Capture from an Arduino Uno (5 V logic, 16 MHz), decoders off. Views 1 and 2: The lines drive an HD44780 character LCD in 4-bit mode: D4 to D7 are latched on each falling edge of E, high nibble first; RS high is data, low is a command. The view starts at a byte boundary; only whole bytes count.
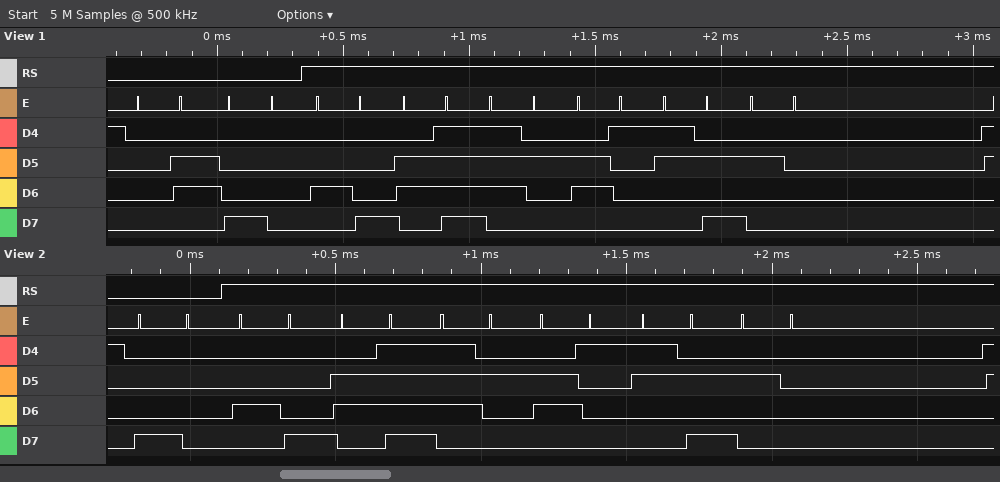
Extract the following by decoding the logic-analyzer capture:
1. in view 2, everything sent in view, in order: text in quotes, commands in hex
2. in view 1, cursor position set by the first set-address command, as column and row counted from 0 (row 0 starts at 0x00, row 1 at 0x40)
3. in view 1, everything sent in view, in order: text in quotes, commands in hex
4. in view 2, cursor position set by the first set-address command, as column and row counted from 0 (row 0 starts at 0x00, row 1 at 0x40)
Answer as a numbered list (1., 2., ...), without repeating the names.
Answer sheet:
1. 0x80 "Hora: "
2. column 0, row 0
3. 0x06 0x80 "Hora: "
4. column 0, row 0
